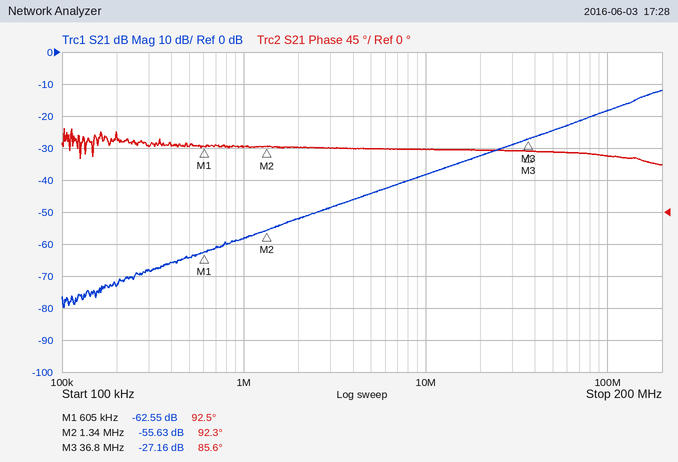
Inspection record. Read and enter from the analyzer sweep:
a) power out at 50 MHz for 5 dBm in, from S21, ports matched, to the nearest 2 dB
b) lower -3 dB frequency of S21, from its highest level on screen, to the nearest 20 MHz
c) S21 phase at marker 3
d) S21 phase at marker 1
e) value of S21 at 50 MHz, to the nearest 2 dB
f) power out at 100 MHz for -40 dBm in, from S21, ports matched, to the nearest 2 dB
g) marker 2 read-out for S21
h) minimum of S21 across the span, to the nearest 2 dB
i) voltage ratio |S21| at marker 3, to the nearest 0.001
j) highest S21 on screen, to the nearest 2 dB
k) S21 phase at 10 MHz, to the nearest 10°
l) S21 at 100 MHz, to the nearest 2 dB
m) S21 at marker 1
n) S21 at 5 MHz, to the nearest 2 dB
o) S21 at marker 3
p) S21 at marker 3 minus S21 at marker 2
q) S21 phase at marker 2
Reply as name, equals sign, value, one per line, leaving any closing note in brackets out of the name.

power out at 50 MHz for 5 dBm in, from S21, ports matched, to the nearest 2 dB = -20 dBm
lower -3 dB frequency of S21, from its highest level on screen, to the nearest 20 MHz = 140 MHz
S21 phase at marker 3 = 85.6°
S21 phase at marker 1 = 92.5°
value of S21 at 50 MHz, to the nearest 2 dB = -24 dB
power out at 100 MHz for -40 dBm in, from S21, ports matched, to the nearest 2 dB = -58 dBm
marker 2 read-out for S21 = -55.63 dB
minimum of S21 across the span, to the nearest 2 dB = -80 dB
voltage ratio |S21| at marker 3, to the nearest 0.001 = 0.044
highest S21 on screen, to the nearest 2 dB = -12 dB
S21 phase at 10 MHz, to the nearest 10° = 90°
S21 at 100 MHz, to the nearest 2 dB = -18 dB
S21 at marker 1 = -62.55 dB
S21 at 5 MHz, to the nearest 2 dB = -44 dB
S21 at marker 3 = -27.16 dB
S21 at marker 3 minus S21 at marker 2 = 28.47 dB
S21 phase at marker 2 = 92.3°
